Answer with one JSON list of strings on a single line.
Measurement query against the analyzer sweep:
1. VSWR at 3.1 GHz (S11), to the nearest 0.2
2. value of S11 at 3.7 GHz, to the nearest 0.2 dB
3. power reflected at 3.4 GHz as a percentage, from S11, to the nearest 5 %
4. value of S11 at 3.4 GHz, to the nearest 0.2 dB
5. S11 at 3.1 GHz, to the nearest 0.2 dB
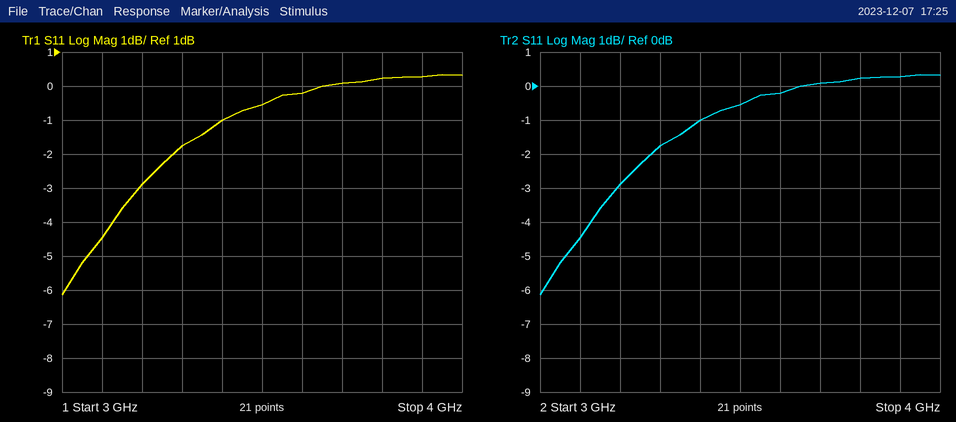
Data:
["4.0", "0.0 dB", "80 %", "-1.0 dB", "-4.4 dB"]
